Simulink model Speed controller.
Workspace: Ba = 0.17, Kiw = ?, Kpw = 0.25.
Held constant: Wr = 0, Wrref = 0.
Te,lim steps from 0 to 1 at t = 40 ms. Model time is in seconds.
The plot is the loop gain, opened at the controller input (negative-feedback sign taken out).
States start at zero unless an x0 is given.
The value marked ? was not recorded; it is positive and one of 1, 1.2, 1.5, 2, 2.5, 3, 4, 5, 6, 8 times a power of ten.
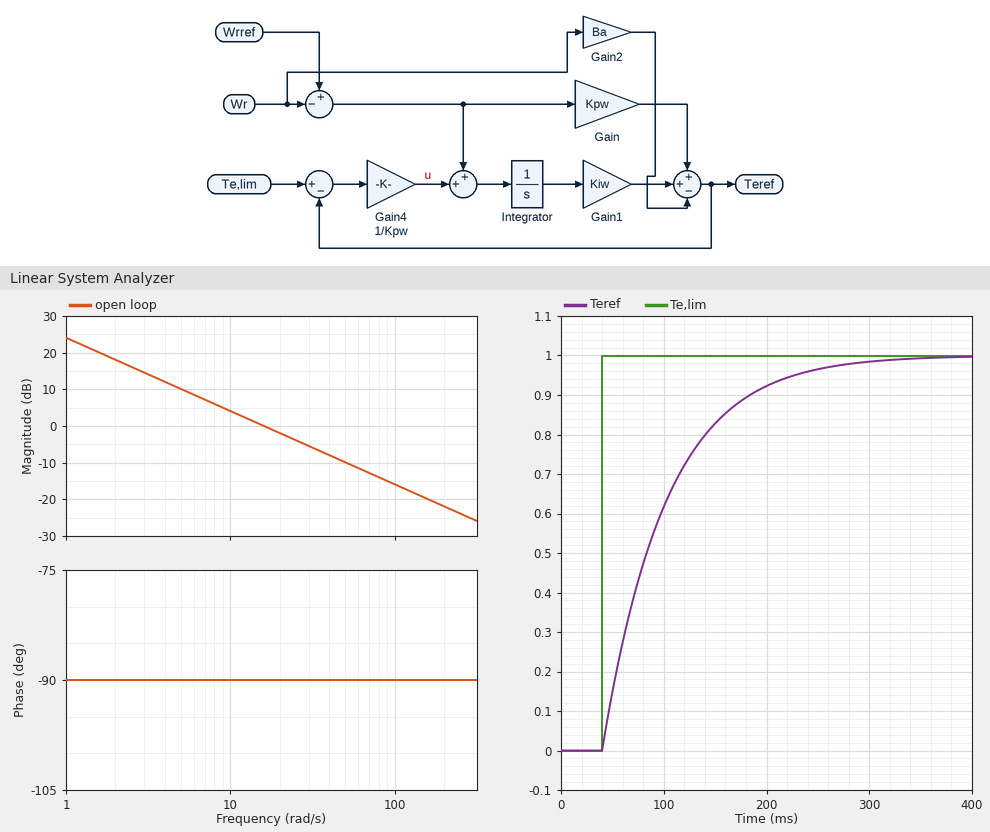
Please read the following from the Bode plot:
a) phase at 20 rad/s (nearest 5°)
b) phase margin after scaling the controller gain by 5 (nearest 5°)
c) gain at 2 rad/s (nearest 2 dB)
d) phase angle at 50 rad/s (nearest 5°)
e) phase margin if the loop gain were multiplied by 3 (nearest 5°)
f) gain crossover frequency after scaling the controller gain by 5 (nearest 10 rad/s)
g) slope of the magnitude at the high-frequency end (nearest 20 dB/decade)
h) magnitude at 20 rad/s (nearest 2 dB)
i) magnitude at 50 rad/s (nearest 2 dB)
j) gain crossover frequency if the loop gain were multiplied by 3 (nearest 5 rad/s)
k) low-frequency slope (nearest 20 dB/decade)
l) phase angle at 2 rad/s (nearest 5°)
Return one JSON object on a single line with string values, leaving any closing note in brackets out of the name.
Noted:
{"phase at 20 rad/s": "-90°", "phase margin after scaling the controller gain by 5": "90°", "gain at 2 rad/s": "18 dB", "phase angle at 50 rad/s": "-90°", "phase margin if the loop gain were multiplied by 3": "90°", "gain crossover frequency after scaling the controller gain by 5": "80 rad/s", "slope of the magnitude at the high-frequency end": "-20 dB/decade", "magnitude at 20 rad/s": "-2 dB", "magnitude at 50 rad/s": "-10 dB", "gain crossover frequency if the loop gain were multiplied by 3": "50 rad/s", "low-frequency slope": "-20 dB/decade", "phase angle at 2 rad/s": "-90°"}
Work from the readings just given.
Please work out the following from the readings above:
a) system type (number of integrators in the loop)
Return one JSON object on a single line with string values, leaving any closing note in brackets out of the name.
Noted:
{"system type": "1"}
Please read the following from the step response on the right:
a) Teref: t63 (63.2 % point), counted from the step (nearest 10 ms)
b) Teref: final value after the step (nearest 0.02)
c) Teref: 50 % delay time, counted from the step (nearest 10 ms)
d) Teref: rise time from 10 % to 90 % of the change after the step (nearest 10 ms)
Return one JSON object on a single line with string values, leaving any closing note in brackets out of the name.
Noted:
{"Teref: t63 (63.2 % point), counted from the step": "60 ms", "Teref: final value after the step": "1.00", "Teref: 50 % delay time, counted from the step": "40 ms", "Teref: rise time from 10 % to 90 % of the change after the step": "140 ms"}
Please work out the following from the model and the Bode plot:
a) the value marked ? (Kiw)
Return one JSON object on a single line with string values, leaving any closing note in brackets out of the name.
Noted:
{"the value marked ?": "4"}
